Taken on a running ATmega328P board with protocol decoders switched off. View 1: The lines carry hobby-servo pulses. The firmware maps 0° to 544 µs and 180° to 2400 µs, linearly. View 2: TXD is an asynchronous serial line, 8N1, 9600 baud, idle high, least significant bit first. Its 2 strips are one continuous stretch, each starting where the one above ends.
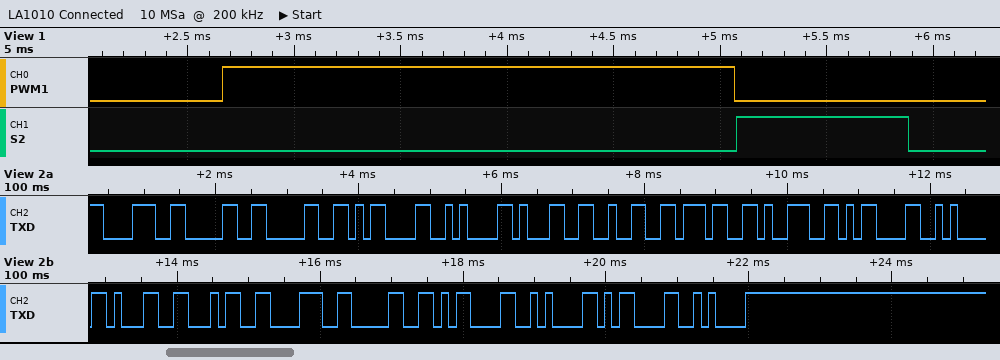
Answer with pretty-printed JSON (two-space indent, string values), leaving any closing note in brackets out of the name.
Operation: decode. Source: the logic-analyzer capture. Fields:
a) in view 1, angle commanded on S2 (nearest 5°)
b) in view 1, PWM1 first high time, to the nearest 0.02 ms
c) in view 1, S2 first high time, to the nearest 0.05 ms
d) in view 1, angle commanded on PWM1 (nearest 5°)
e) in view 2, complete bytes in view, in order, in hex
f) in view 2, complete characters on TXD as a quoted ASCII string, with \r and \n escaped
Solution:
{
  "in view 1, angle commanded on S2": "25°",
  "in view 1, PWM1 first high time, to the nearest 0.02 ms": "2.40 ms",
  "in view 1, S2 first high time, to the nearest 0.05 ms": "0.80 ms",
  "in view 1, angle commanded on PWM1": "180°",
  "in view 2, complete bytes in view, in order, in hex": "38 30 30 0D 0A 31 32 37 39 0D 0A 31 34 38 30 0D 0A 0D 0A",
  "in view 2, complete characters on TXD as a quoted ASCII string, with \\r and \\n escaped": "\"800\\r\\n1279\\r\\n1480\\r\\n\\r\\n\""
}
